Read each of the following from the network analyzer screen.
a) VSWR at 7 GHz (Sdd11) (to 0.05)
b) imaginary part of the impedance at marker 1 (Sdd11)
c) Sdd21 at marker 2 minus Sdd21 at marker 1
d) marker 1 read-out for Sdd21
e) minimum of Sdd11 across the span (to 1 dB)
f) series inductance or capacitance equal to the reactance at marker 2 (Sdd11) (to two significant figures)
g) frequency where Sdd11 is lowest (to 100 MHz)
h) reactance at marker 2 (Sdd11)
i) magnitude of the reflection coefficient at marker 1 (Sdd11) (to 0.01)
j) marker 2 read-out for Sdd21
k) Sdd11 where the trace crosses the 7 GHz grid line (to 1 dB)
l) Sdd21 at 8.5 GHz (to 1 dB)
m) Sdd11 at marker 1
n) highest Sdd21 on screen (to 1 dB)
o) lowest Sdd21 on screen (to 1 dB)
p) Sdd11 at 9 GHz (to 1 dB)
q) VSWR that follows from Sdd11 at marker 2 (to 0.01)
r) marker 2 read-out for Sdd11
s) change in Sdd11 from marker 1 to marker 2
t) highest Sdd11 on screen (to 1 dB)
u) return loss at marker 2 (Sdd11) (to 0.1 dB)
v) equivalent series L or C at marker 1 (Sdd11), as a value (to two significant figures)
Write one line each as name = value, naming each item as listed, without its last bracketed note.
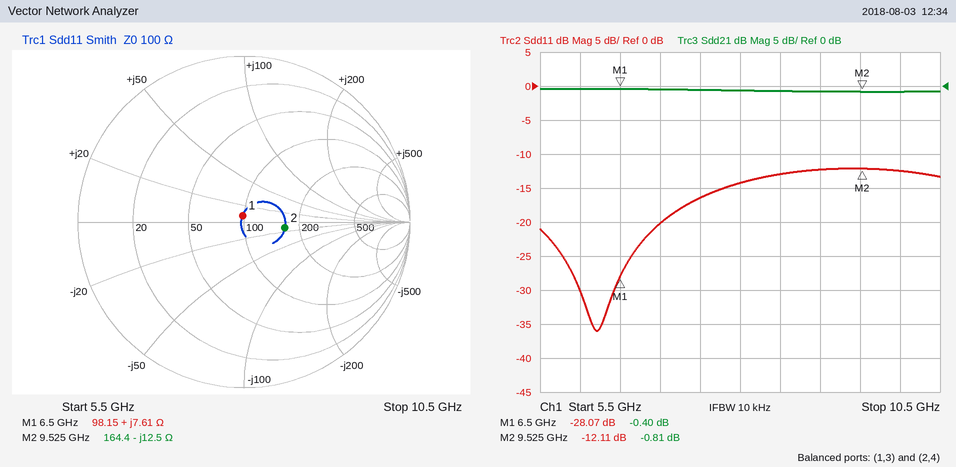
VSWR at 7 GHz (Sdd11) = 1.20
imaginary part of the impedance at marker 1 = +7.61 Ω
Sdd21 at marker 2 minus Sdd21 at marker 1 = -0.41 dB
marker 1 read-out for Sdd21 = -0.40 dB
minimum of Sdd11 across the span = -36 dB
series inductance or capacitance equal to the reactance at marker 2 (Sdd11) = 1.3 pF
frequency where Sdd11 is lowest = 6.2 GHz
reactance at marker 2 = -12.5 Ω
magnitude of the reflection coefficient at marker 1 (Sdd11) = 0.04
marker 2 read-out for Sdd21 = -0.81 dB
Sdd11 where the trace crosses the 7 GHz grid line = -20 dB
Sdd21 at 8.5 GHz = -1 dB
Sdd11 at marker 1 = -28.07 dB
highest Sdd21 on screen = 0 dB
lowest Sdd21 on screen = -1 dB
Sdd11 at 9 GHz = -12 dB
VSWR that follows from Sdd11 at marker 2 = 1.66
marker 2 read-out for Sdd11 = -12.11 dB
change in Sdd11 from marker 1 to marker 2 = 15.96 dB
highest Sdd11 on screen = -12 dB
return loss at marker 2 (Sdd11) = 12.1 dB
equivalent series L or C at marker 1 (Sdd11), as a value = 190 pH
